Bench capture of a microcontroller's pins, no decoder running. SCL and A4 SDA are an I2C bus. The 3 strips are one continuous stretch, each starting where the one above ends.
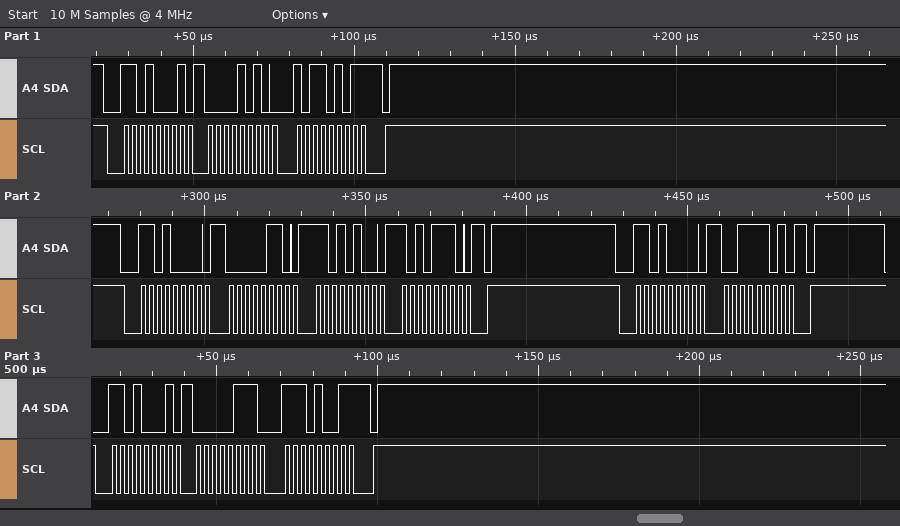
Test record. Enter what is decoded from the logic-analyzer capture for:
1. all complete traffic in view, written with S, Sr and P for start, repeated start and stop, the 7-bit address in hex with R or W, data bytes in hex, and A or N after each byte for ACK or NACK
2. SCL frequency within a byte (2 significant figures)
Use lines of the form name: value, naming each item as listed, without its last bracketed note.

all complete traffic in view, written with S, Sr and P for start, repeated start and stop, the 7-bit address in hex with R or W, data bytes in hex, and A or N after each byte for ACK or NACK: S 68R A 0A A B5 N P S 68W A 06 A D4 A AE A P S 68W A 3D A P S 68R A 07 A E9 N P
SCL frequency within a byte: 400 kHz
